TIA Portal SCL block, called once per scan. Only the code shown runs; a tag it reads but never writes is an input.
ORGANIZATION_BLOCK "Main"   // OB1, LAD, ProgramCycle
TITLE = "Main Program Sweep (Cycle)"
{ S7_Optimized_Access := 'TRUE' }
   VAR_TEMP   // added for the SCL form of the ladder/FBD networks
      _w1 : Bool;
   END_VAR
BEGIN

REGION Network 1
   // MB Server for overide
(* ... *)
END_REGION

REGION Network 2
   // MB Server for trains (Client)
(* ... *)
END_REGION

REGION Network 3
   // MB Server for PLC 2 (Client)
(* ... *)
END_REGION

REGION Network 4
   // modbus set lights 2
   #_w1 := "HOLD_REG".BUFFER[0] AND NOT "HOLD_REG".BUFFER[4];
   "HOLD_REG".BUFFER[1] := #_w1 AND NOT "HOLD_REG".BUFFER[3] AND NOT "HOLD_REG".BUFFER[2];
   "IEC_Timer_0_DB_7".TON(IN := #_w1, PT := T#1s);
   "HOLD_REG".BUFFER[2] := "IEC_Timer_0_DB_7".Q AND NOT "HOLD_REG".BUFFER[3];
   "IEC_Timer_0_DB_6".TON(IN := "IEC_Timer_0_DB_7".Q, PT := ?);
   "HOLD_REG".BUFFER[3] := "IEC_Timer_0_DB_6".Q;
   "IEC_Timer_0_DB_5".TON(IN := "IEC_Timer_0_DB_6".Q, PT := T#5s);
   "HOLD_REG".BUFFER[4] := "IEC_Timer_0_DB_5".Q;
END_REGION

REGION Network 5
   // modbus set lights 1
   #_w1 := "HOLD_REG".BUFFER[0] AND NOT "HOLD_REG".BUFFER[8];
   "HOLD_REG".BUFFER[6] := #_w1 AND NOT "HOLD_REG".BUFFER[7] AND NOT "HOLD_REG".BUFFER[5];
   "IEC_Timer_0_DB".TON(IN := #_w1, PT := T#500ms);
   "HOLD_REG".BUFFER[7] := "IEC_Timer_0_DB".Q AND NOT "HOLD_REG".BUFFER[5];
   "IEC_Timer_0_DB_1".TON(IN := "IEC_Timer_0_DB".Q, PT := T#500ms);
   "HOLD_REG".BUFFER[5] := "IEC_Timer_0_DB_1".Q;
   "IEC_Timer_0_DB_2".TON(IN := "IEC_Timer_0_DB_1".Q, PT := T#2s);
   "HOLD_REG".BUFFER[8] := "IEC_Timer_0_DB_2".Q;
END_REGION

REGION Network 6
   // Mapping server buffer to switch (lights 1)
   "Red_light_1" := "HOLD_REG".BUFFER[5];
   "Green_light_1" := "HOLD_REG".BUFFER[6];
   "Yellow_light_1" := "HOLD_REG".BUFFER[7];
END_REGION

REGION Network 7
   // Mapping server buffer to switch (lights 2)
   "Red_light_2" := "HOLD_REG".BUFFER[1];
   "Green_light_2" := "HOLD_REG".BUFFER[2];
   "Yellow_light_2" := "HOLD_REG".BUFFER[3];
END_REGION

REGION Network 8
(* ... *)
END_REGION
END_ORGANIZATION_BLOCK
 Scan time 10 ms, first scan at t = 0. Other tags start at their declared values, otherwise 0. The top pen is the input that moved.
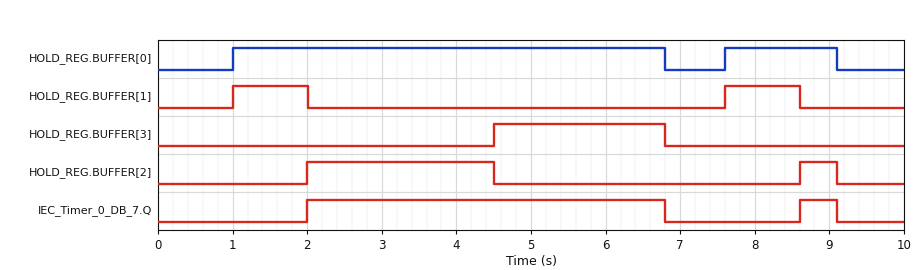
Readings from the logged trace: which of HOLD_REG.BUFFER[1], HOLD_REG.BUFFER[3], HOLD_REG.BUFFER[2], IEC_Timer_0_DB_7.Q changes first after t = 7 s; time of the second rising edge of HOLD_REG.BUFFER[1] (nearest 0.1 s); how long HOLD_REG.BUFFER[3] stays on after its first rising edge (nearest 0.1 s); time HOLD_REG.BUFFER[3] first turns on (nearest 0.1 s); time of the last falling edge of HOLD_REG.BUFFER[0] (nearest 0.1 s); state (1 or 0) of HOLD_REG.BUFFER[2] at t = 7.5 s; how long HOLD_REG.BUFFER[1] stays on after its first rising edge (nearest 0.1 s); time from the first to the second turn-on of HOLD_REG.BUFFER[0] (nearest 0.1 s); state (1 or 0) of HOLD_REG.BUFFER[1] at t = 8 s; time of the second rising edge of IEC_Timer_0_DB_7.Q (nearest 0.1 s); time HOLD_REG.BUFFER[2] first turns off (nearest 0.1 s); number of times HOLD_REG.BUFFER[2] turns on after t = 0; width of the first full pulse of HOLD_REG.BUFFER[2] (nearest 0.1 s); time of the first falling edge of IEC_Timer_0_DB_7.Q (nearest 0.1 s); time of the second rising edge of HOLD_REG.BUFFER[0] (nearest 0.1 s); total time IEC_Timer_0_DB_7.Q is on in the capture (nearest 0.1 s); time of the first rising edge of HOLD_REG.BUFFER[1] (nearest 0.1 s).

HOLD_REG.BUFFER[1]
7.6 s
2.3 s
4.5 s
9.1 s
0
1.0 s
6.6 s
1
8.6 s
4.5 s
2
2.5 s
6.8 s
7.6 s
5.3 s
1.0 s
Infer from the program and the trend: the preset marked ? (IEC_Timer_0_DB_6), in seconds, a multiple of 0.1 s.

2.5 s
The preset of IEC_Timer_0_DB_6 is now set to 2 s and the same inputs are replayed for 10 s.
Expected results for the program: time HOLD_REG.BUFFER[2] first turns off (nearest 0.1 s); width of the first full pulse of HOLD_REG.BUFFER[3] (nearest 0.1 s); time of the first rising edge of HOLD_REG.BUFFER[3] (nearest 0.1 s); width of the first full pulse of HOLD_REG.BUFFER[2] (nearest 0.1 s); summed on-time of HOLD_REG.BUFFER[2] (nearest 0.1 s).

4.0 s
2.8 s
4.0 s
2.0 s
2.5 s
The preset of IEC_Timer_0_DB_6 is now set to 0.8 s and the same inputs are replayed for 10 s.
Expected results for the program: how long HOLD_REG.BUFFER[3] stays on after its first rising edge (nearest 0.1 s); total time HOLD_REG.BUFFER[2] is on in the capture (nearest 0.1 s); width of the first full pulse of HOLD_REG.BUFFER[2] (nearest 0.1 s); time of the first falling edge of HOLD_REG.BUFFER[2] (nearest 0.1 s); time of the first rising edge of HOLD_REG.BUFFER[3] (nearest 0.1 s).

4.0 s
1.3 s
0.8 s
2.8 s
2.8 s
